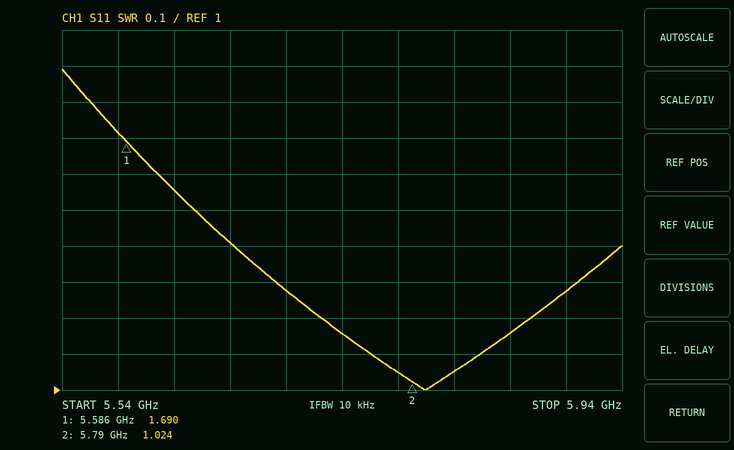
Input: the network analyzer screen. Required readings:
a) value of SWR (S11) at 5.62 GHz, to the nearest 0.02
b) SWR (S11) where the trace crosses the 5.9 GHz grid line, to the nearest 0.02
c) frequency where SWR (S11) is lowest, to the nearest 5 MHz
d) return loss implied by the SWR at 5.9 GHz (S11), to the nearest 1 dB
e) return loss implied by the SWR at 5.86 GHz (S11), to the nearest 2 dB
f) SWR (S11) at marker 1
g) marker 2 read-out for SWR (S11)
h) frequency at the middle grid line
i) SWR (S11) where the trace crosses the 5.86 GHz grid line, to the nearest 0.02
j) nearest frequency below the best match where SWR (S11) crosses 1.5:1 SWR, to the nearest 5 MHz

1.56
1.28
5.800 GHz
18 dB
22 dB
1.690
1.024
5.74 GHz
1.16
5.635 GHz
